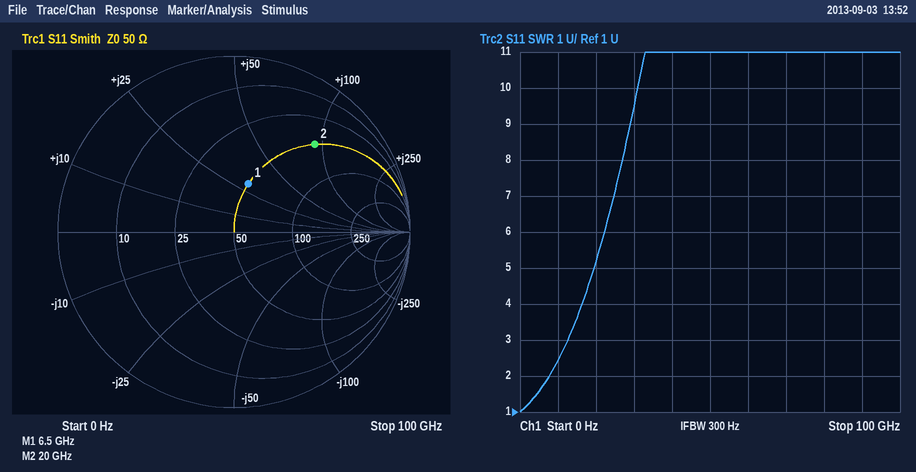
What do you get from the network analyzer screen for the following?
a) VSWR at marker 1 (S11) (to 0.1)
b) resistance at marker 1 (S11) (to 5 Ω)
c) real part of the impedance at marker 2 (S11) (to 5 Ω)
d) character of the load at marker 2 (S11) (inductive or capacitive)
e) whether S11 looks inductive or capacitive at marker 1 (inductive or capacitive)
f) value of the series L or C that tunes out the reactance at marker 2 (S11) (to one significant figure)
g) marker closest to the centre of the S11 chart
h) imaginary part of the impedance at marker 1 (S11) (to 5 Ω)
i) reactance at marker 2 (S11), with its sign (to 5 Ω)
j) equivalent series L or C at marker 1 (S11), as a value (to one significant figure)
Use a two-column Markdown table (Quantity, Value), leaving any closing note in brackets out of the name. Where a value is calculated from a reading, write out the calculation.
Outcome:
| Quantity | Value |
|---|---|
| VSWR at marker 1 (S11) | 1.8 |
| resistance at marker 1 (S11) | 50 Ω |
| real part of the impedance at marker 2 (S11) | 50 Ω |
| character of the load at marker 2 (S11) | inductive |
| whether S11 looks inductive or capacitive at marker 1 | inductive |
| value of the series L or C that tunes out the reactance at marker 2 (S11) | C = 1/(2π × 20 GHz × 90 Ω) ≈ 88.4 fF, so 90 fF to one significant figure |
| marker closest to the centre of the S11 chart | marker 1 |
| imaginary part of the impedance at marker 1 (S11) | +30 Ω |
| reactance at marker 2 (S11), with its sign | +90 Ω |
| equivalent series L or C at marker 1 (S11), as a value | L = 30 Ω/(2π × 6.5 GHz) ≈ 735 pH, so 700 pH to one significant figure |
